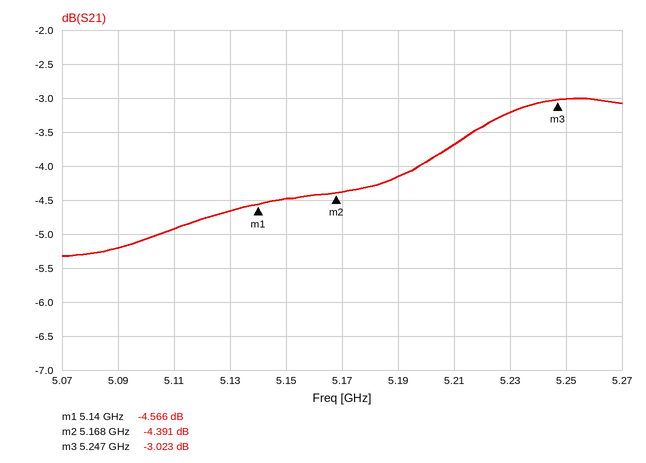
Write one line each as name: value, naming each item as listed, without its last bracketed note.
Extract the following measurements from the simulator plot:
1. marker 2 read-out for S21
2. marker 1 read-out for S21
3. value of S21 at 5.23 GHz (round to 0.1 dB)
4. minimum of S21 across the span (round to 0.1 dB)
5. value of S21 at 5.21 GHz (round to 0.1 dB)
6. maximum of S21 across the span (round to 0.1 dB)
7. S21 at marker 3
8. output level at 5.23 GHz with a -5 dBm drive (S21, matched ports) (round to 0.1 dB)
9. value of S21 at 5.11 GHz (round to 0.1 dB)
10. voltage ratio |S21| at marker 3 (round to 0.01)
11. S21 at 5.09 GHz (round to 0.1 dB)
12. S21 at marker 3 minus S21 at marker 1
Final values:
marker 2 read-out for S21: -4.391 dB
marker 1 read-out for S21: -4.566 dB
value of S21 at 5.23 GHz: -3.2 dB
minimum of S21 across the span: -5.3 dB
value of S21 at 5.21 GHz: -3.7 dB
maximum of S21 across the span: -3.0 dB
S21 at marker 3: -3.023 dB
output level at 5.23 GHz with a -5 dBm drive (S21, matched ports): -8.2 dBm
value of S21 at 5.11 GHz: -4.9 dB
voltage ratio |S21| at marker 3: 0.71
S21 at 5.09 GHz: -5.2 dB
S21 at marker 3 minus S21 at marker 1: 1.543 dB
